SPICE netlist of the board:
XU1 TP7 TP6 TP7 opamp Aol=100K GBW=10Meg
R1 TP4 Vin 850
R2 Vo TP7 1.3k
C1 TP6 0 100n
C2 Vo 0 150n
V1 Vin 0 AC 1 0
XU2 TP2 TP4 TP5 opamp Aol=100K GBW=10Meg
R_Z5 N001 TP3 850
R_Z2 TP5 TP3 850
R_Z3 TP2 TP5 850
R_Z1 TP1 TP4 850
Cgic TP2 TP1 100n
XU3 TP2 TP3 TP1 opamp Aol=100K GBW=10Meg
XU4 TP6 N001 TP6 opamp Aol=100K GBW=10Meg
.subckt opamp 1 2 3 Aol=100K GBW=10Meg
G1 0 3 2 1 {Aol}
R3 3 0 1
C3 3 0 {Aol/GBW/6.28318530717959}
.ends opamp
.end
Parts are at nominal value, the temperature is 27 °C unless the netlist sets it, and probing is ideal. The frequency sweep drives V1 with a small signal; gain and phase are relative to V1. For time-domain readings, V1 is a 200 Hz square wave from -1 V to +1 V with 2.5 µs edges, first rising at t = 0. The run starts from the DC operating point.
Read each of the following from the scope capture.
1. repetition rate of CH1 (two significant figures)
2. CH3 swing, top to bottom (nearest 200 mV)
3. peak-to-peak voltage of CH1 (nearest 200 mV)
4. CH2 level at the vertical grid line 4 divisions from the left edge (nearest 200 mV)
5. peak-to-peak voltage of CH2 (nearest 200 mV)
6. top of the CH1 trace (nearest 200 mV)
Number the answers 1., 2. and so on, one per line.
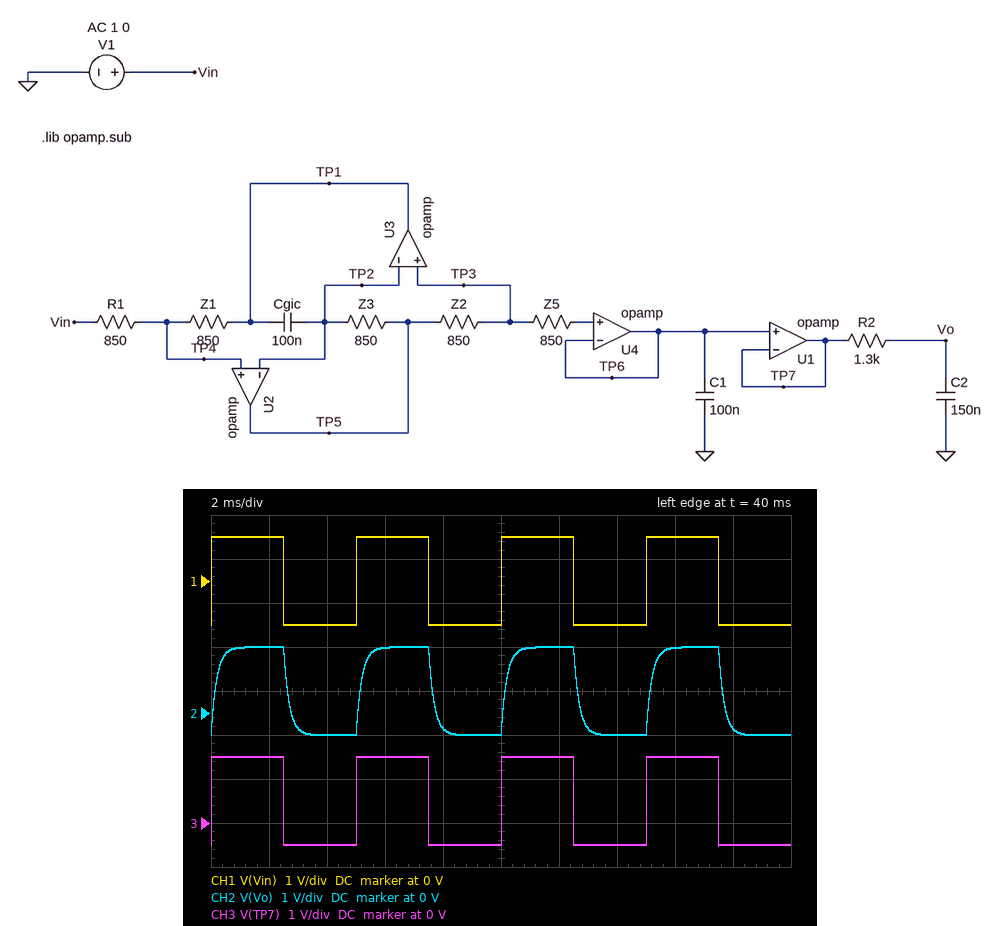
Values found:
1. 200 Hz
2. 2.0 V
3. 2.0 V
4. -400 mV
5. 2.0 V
6. 1.0 V
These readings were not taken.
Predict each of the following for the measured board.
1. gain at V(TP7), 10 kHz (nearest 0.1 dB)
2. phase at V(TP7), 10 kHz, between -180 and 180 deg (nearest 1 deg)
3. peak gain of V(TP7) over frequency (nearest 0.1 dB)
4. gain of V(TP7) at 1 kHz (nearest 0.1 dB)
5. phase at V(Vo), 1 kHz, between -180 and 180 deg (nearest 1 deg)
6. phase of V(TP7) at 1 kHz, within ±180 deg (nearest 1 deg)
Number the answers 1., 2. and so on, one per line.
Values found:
1. 0 dB
2. 0 deg
3. 0 dB
4. 0 dB
5. -51 deg
6. 0 deg
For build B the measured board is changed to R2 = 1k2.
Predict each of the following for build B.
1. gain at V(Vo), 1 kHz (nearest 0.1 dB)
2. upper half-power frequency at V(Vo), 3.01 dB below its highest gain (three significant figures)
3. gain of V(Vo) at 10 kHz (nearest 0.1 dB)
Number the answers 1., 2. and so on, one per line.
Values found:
1. -3.6 dB
2. 884 Hz
3. -21.1 dB
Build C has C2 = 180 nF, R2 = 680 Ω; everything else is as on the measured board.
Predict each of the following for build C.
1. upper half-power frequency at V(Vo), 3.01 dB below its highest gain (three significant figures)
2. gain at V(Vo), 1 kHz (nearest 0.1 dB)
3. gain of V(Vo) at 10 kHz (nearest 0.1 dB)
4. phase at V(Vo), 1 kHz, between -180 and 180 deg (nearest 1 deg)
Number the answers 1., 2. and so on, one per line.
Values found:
1. 1.30 kHz
2. -2.0 dB
3. -17.8 dB
4. -38 deg
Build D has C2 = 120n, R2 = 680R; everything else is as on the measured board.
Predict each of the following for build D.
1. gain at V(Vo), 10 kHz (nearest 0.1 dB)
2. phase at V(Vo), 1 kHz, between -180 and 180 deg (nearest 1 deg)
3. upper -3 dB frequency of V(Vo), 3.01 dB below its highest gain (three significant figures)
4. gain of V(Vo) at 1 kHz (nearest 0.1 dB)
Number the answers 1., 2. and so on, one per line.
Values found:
1. -14.4 dB
2. -27 deg
3. 1.95 kHz
4. -1.0 dB
